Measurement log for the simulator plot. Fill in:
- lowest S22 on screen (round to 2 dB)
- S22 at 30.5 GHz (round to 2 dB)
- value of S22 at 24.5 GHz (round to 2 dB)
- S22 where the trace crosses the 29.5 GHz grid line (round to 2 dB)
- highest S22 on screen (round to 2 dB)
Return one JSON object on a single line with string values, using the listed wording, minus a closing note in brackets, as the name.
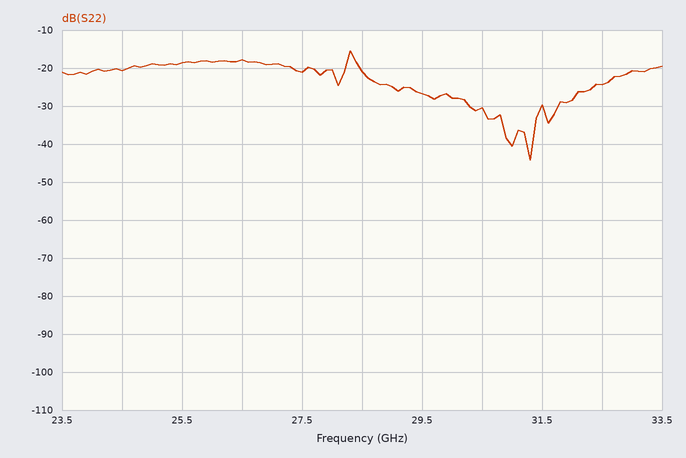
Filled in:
{"lowest S22 on screen": "-44 dB", "S22 at 30.5 GHz": "-30 dB", "value of S22 at 24.5 GHz": "-20 dB", "S22 where the trace crosses the 29.5 GHz grid line": "-26 dB", "highest S22 on screen": "-16 dB"}
